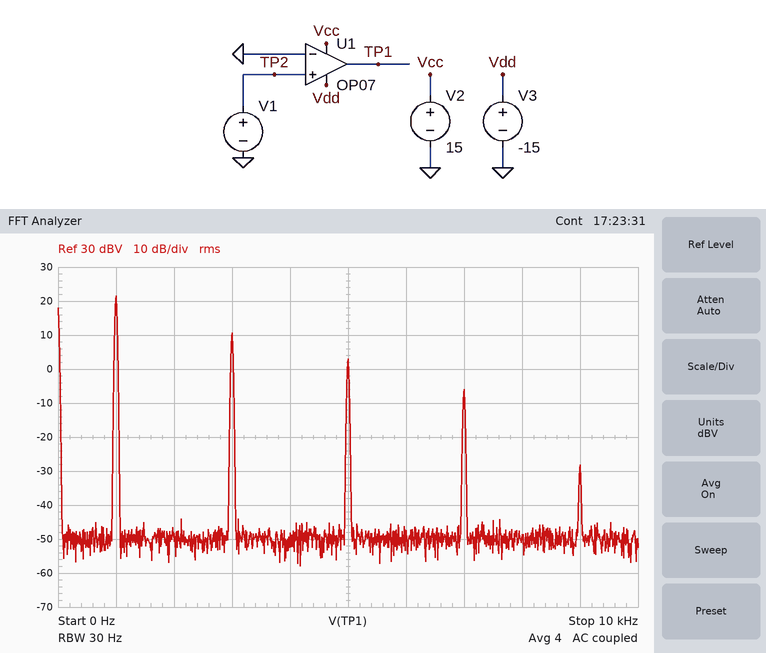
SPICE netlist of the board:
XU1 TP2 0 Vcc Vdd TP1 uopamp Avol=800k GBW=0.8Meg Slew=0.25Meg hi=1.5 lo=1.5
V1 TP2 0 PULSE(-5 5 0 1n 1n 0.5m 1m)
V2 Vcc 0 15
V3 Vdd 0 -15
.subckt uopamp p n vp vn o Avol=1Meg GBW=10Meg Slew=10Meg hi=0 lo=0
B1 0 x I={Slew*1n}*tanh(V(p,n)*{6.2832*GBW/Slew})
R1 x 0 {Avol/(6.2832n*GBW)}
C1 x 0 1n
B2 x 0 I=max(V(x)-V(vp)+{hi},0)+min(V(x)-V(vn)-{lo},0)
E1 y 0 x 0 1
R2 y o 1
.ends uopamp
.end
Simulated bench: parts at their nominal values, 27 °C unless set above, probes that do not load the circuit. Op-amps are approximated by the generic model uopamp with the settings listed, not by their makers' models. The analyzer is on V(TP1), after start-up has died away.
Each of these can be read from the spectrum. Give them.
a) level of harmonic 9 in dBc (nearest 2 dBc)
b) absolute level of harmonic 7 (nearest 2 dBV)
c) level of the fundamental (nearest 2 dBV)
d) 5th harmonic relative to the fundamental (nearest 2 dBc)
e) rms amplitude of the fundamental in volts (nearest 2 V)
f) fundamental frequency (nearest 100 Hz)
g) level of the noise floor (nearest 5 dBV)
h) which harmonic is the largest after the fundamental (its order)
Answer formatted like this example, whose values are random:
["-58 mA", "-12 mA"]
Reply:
["-50 dBc", "-6 dBV", "22 dBV", "-18 dBc", "12 V", "1.0 kHz", "-50 dBV", "3"]
